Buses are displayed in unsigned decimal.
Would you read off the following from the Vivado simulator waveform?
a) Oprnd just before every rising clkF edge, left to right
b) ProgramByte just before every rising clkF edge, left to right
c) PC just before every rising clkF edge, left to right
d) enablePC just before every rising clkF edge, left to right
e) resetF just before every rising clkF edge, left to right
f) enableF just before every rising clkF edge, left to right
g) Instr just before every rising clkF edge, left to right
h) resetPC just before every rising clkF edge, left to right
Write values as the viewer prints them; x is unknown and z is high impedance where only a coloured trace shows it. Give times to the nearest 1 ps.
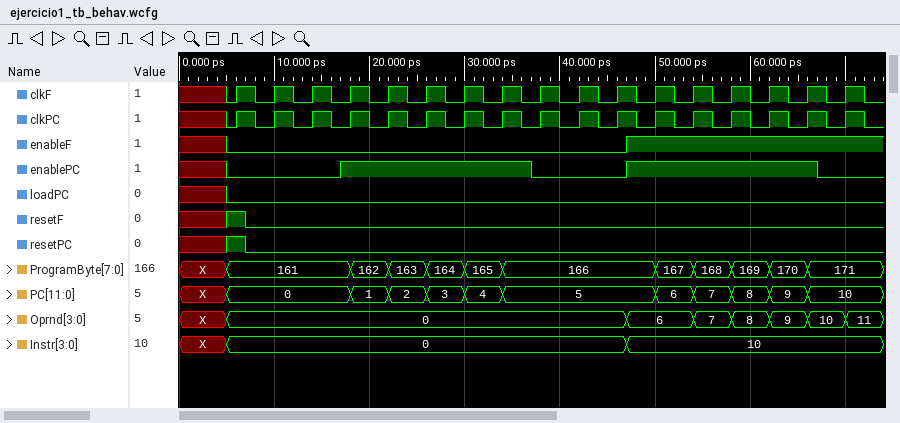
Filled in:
0, 0, 0, 0, 0, 0, 0, 0, 0, 0, 0, 6, 6, 7, 8, 9, 10
161, 161, 161, 161, 162, 163, 164, 165, 166, 166, 166, 166, 167, 168, 169, 170, 171
0, 0, 0, 0, 1, 2, 3, 4, 5, 5, 5, 5, 6, 7, 8, 9, 10
0 0 0 1 1 1 1 1 0 0 0 1 1 1 1 1 0
1 0 0 0 0 0 0 0 0 0 0 0 0 0 0 0 0
0 0 0 0 0 0 0 0 0 0 0 1 1 1 1 1 1
0, 0, 0, 0, 0, 0, 0, 0, 0, 0, 0, 10, 10, 10, 10, 10, 10
1 0 0 0 0 0 0 0 0 0 0 0 0 0 0 0 0
